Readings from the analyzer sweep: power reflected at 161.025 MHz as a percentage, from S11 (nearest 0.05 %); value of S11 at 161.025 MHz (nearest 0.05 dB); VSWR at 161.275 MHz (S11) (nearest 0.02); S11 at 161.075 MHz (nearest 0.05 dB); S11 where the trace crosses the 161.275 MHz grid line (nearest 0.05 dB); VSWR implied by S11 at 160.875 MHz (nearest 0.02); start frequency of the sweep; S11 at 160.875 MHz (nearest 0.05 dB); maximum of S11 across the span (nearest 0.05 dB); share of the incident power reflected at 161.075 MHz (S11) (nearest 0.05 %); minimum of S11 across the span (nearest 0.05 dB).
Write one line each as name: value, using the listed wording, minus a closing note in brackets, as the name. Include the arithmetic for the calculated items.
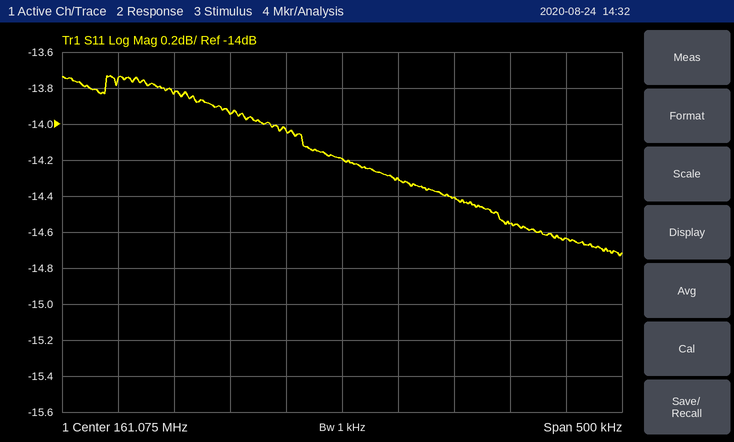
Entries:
power reflected at 161.025 MHz as a percentage, from S11: 10^(-14.05/10) ≈ 3.94 %, so 3.95 % to the nearest 0.05 %
value of S11 at 161.025 MHz: -14.05 dB
VSWR at 161.275 MHz (S11): |Γ| = 10^(-14.65/20) = 0.1851; VSWR = (1 + 0.1851)/(1 − 0.1851) ≈ 1.45, so 1.46 to the nearest 0.02
S11 at 161.075 MHz: -14.20 dB
S11 where the trace crosses the 161.275 MHz grid line: -14.65 dB
VSWR implied by S11 at 160.875 MHz: |Γ| = 10^(-13.75/20) = 0.2054; VSWR = (1 + 0.2054)/(1 − 0.2054) ≈ 1.52
start frequency of the sweep: 160.825 MHz
S11 at 160.875 MHz: -13.75 dB
maximum of S11 across the span: -13.75 dB
share of the incident power reflected at 161.075 MHz (S11): 10^(-14.2/10) ≈ 3.80 %
minimum of S11 across the span: -14.75 dB
